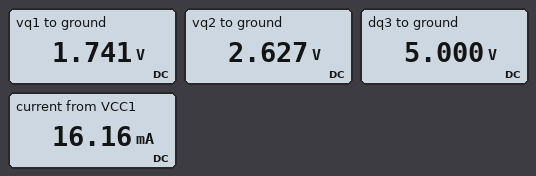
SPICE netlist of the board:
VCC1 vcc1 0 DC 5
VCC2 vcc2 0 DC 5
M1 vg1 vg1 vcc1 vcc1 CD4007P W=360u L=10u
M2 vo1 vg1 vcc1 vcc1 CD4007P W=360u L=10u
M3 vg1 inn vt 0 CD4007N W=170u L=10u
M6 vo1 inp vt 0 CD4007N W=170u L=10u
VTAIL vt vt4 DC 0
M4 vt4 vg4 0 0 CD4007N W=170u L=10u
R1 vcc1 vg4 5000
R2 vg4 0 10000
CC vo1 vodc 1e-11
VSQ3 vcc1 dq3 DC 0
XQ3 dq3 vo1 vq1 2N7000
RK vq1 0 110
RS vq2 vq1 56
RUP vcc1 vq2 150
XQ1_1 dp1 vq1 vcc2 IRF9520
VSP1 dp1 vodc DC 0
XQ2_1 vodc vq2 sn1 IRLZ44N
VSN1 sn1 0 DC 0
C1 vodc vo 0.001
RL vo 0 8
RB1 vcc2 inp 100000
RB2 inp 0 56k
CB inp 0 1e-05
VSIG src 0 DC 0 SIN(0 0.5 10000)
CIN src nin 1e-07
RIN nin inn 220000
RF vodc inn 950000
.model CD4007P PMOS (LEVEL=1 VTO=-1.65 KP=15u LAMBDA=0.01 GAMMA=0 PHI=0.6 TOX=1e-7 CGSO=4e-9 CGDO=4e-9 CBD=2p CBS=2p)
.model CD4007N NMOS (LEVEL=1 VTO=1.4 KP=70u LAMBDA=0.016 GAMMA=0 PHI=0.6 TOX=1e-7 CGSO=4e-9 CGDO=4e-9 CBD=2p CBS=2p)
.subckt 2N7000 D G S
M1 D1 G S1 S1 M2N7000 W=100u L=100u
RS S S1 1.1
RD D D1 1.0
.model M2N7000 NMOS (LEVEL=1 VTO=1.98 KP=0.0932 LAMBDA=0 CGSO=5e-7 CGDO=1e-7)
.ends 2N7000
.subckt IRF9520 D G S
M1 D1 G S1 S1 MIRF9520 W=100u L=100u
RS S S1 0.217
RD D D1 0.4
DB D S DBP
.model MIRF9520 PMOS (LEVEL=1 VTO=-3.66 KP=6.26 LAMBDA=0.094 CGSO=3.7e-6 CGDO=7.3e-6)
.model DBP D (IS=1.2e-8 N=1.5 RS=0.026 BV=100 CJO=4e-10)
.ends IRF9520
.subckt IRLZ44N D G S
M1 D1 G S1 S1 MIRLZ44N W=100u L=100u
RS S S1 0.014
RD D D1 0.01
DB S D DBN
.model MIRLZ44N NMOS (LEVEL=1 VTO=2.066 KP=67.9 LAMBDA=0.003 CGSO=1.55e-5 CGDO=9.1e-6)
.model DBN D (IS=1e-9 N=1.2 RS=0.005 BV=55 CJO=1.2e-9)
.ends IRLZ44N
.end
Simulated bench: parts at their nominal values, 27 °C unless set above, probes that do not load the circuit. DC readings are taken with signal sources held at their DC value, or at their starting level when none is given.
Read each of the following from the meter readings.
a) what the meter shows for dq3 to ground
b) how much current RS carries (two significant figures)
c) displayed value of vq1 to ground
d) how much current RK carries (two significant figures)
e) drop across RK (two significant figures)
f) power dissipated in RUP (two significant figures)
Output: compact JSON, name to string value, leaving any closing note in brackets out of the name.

{"what the meter shows for dq3 to ground": "5.000 V", "how much current RS carries": "16 mA", "displayed value of vq1 to ground": "1.741 V", "how much current RK carries": "16 mA", "drop across RK": "1.7 V", "power dissipated in RUP": "38 mW"}
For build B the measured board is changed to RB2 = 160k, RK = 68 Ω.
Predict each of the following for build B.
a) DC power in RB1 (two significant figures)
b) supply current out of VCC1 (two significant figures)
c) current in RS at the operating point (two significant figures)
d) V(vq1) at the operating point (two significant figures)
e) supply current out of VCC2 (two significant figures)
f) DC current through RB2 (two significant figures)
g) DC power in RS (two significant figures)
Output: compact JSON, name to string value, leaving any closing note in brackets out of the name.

{"DC power in RB1": "37 µW", "supply current out of VCC1": "19 mA", "current in RS at the operating point": "18 mA", "V(vq1) at the operating point": "1.2 V", "supply current out of VCC2": "38 mA", "DC current through RB2": "19 µA", "DC power in RS": "19 mW"}
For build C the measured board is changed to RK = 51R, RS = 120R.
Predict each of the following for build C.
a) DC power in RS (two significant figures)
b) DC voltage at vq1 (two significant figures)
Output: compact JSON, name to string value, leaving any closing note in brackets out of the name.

{"DC power in RS": "29 mW", "DC voltage at vq1": "790 mV"}
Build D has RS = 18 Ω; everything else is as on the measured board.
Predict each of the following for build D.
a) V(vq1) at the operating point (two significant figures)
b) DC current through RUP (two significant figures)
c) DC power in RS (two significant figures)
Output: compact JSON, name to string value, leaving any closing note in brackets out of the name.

{"V(vq1) at the operating point": "2.0 V", "DC current through RUP": "18 mA", "DC power in RS": "5.8 mW"}
